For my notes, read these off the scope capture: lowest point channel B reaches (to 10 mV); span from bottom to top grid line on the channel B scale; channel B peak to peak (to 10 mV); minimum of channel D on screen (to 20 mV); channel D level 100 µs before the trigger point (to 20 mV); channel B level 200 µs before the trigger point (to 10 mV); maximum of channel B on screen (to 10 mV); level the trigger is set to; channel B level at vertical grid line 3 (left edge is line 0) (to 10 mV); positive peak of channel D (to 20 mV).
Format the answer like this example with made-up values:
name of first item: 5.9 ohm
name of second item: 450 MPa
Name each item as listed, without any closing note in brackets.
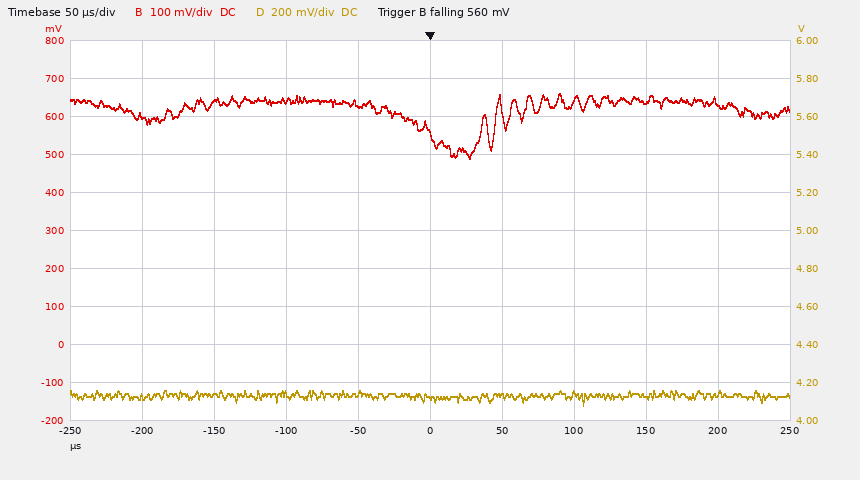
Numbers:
lowest point channel B reaches: 490 mV
span from bottom to top grid line on the channel B scale: 1 V
channel B peak to peak: 170 mV
minimum of channel D on screen: 4.08 V
channel D level 100 µs before the trigger point: 4.14 V
channel B level 200 µs before the trigger point: 600 mV
maximum of channel B on screen: 660 mV
level the trigger is set to: 560 mV
channel B level at vertical grid line 3 (left edge is line 0): 640 mV
positive peak of channel D: 4.16 V
